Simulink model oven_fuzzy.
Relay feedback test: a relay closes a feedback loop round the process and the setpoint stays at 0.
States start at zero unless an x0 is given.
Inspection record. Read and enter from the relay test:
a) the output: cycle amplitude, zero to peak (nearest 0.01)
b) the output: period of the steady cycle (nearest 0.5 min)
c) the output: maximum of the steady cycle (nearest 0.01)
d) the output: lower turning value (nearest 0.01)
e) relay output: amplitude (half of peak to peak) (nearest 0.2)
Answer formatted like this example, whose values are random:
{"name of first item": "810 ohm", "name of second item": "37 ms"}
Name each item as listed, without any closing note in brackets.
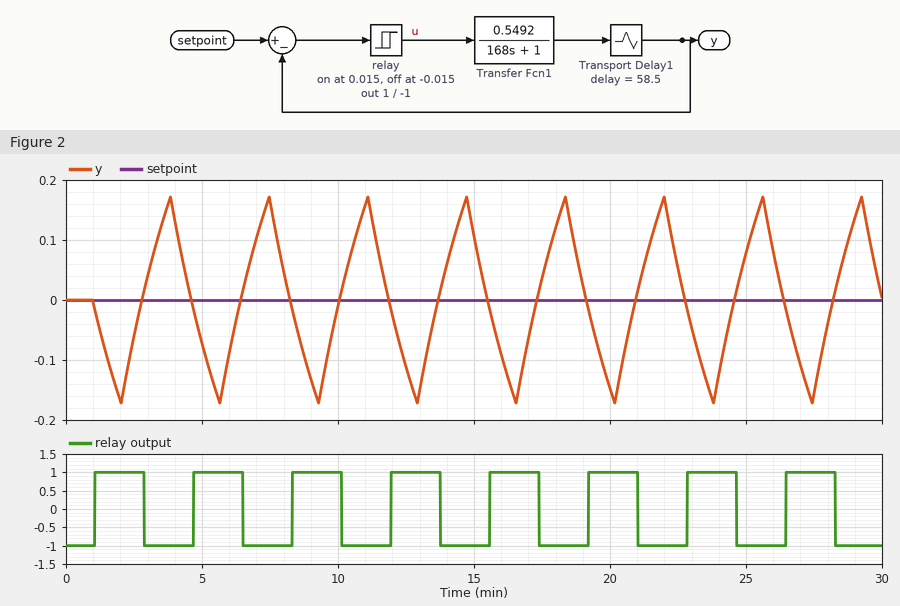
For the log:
{"the output: cycle amplitude, zero to peak": "0.17", "the output: period of the steady cycle": "3.5 min", "the output: maximum of the steady cycle": "0.17", "the output: lower turning value": "-0.17", "relay output: amplitude (half of peak to peak)": "1.0"}
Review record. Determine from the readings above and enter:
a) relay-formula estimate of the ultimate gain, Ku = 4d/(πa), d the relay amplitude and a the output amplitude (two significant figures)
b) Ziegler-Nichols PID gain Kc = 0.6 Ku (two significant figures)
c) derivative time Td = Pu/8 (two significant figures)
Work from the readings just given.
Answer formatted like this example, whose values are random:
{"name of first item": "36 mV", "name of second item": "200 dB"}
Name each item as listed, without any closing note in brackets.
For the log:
{"relay-formula estimate of the ultimate gain, Ku = 4d/(πa), d the relay amplitude and a the output amplitude": "7.5", "Ziegler-Nichols PID gain Kc = 0.6 Ku": "4.5", "derivative time Td = Pu/8": "0.44 min"}
